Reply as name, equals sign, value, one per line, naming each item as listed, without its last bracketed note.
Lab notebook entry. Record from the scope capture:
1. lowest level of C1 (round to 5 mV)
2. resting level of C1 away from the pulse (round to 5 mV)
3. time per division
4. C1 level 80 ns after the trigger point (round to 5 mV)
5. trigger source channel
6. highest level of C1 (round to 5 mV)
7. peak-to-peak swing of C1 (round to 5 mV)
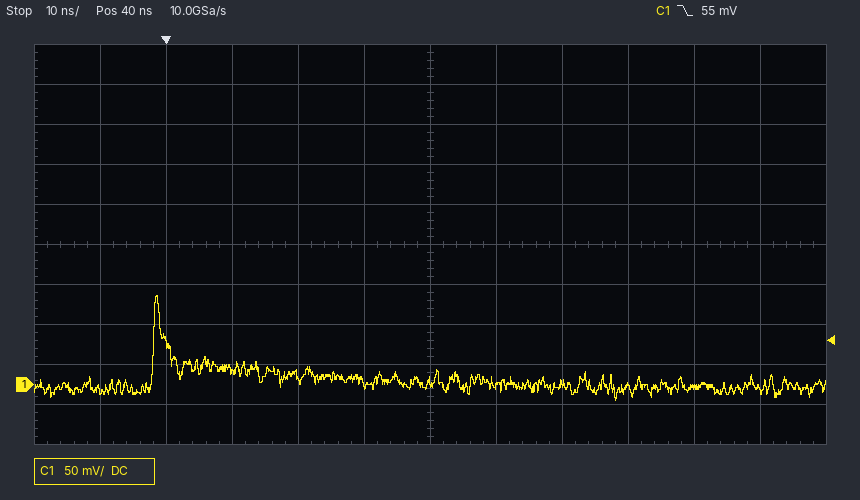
lowest level of C1 = -20 mV
resting level of C1 away from the pulse = 0 mV
time per division = 10 ns
C1 level 80 ns after the trigger point = -5 mV
trigger source channel = C1
highest level of C1 = 110 mV
peak-to-peak swing of C1 = 130 mV
